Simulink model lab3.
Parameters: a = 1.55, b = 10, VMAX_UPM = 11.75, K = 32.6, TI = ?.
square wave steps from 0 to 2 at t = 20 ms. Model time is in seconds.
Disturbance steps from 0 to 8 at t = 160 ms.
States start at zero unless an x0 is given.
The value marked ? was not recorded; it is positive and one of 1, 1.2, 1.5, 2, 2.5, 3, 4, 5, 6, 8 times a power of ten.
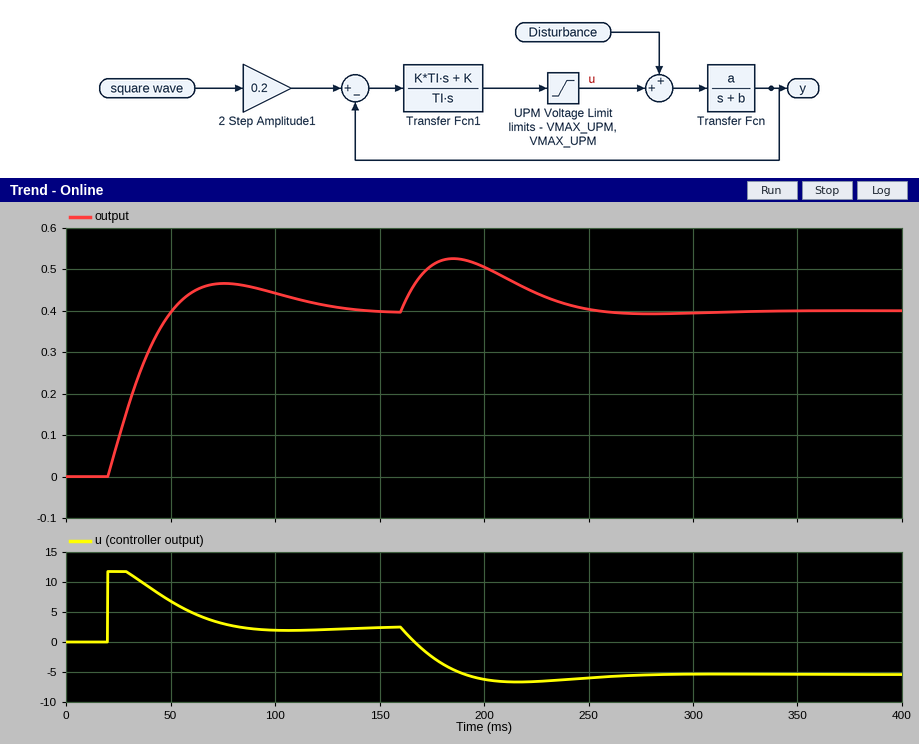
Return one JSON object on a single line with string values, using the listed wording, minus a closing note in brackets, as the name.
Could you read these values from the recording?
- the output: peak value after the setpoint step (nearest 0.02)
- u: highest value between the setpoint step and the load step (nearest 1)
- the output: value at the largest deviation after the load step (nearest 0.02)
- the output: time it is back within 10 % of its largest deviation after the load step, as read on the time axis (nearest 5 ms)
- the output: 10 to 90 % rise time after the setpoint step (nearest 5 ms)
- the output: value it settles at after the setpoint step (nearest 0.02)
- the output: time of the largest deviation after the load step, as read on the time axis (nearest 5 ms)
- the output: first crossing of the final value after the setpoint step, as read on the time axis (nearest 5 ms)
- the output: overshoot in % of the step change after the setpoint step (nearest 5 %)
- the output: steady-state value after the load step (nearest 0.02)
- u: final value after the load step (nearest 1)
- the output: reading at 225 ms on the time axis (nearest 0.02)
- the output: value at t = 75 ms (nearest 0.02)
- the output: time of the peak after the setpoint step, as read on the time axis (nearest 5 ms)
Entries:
{"the output: peak value after the setpoint step": "0.46", "u: highest value between the setpoint step and the load step": "12", "the output: value at the largest deviation after the load step": "0.52", "the output: time it is back within 10 % of its largest deviation after the load step, as read on the time axis": "240 ms", "the output: 10 to 90 % rise time after the setpoint step": "25 ms", "the output: value it settles at after the setpoint step": "0.40", "the output: time of the largest deviation after the load step, as read on the time axis": "185 ms", "the output: first crossing of the final value after the setpoint step, as read on the time axis": "50 ms", "the output: overshoot in % of the step change after the setpoint step": "15 %", "the output: steady-state value after the load step": "0.40", "u: final value after the load step": "-5", "the output: reading at 225 ms on the time axis": "0.44", "the output: value at t = 75 ms": "0.46", "the output: time of the peak after the setpoint step, as read on the time axis": "75 ms"}
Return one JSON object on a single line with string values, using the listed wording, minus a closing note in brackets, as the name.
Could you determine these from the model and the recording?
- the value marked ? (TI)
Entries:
{"the value marked ?": "0.025"}
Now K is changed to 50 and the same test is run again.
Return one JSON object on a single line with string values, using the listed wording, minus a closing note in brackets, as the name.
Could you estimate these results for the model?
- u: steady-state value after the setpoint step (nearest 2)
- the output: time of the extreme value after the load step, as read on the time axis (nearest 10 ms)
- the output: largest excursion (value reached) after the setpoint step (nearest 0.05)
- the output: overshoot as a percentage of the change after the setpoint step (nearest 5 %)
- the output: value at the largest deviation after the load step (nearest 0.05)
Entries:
{"u: steady-state value after the setpoint step": "2", "the output: time of the extreme value after the load step, as read on the time axis": "180 ms", "the output: largest excursion (value reached) after the setpoint step": "0.50", "the output: overshoot as a percentage of the change after the setpoint step": "20 %", "the output: value at the largest deviation after the load step": "0.50"}
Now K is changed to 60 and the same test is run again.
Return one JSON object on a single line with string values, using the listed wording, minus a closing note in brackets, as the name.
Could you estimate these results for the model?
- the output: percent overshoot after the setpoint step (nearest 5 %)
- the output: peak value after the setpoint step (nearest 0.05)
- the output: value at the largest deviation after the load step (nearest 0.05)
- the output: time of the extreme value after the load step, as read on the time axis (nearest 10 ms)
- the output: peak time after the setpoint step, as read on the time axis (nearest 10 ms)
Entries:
{"the output: percent overshoot after the setpoint step": "25 %", "the output: peak value after the setpoint step": "0.50", "the output: value at the largest deviation after the load step": "0.50", "the output: time of the extreme value after the load step, as read on the time axis": "180 ms", "the output: peak time after the setpoint step, as read on the time axis": "60 ms"}
